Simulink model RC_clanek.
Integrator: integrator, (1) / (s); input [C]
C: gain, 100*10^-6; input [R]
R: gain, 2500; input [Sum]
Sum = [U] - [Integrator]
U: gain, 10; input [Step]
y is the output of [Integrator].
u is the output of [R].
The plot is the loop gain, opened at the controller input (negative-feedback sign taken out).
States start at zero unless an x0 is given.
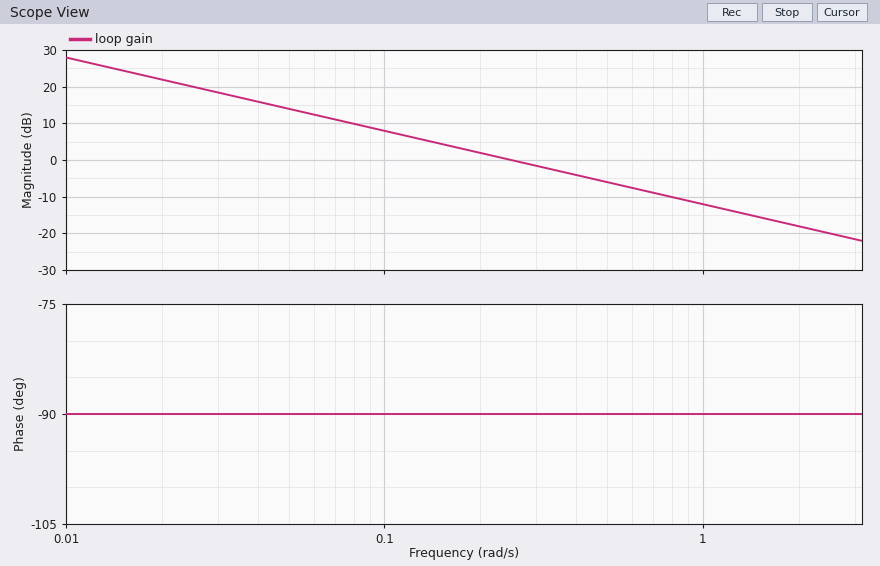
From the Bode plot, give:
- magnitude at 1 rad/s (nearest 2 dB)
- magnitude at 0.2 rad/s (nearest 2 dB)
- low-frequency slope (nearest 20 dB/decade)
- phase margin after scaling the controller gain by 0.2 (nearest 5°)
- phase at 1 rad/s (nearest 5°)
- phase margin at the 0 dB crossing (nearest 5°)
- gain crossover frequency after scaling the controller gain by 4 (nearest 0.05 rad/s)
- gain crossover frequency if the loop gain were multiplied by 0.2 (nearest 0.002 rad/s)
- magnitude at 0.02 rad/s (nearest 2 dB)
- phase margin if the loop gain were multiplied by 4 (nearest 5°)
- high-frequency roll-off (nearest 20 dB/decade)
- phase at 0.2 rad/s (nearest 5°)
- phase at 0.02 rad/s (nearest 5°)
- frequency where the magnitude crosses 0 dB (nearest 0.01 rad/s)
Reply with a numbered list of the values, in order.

1. -12 dB
2. 2 dB
3. -20 dB/decade
4. 90°
5. -90°
6. 90°
7. 1.00 rad/s
8. 0.050 rad/s
9. 22 dB
10. 90°
11. -20 dB/decade
12. -90°
13. -90°
14. 0.25 rad/s
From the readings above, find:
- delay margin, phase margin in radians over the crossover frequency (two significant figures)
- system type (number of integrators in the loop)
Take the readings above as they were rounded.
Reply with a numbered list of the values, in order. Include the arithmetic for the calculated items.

1. 90 × π / 180 / 0.25 = 6.3 s
2. 1
